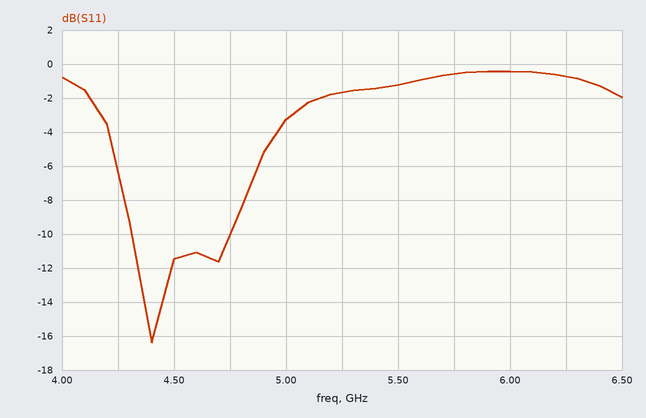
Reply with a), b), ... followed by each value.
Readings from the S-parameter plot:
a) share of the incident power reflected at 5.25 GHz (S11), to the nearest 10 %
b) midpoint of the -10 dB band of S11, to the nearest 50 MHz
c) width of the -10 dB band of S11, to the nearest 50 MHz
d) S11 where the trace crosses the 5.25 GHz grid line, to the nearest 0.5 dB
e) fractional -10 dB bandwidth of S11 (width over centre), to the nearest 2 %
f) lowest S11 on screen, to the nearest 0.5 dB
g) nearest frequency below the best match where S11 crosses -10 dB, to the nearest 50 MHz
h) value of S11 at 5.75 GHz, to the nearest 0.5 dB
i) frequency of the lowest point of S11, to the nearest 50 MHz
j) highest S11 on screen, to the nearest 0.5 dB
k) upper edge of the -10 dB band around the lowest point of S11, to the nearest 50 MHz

a) 70 %
b) 4.55 GHz
c) 450 MHz
d) -1.5 dB
e) 10 %
f) -16.5 dB
g) 4.30 GHz
h) -0.5 dB
i) 4.40 GHz
j) -0.5 dB
k) 4.75 GHz
